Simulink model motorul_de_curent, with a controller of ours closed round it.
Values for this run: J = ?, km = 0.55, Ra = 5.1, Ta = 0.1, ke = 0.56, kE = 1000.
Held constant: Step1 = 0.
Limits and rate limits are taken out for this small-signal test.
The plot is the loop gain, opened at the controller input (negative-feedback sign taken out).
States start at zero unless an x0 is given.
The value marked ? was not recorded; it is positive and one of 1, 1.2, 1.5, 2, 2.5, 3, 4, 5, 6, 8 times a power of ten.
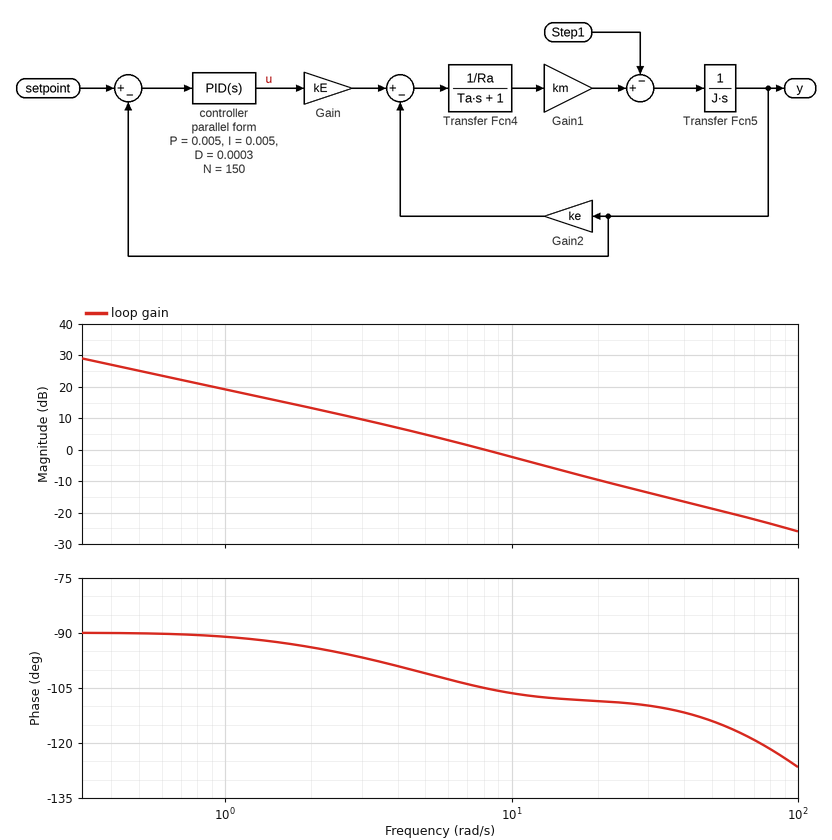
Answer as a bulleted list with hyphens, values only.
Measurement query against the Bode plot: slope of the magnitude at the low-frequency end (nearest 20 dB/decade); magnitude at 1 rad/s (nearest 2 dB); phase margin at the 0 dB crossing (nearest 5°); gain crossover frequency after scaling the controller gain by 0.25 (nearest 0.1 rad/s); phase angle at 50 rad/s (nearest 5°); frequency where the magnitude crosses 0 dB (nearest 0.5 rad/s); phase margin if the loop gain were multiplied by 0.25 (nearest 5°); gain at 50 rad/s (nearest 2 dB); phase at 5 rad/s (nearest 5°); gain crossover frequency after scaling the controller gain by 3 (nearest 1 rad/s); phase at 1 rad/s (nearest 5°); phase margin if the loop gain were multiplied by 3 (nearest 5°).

- -20 dB/decade
- 20 dB
- 75°
- 2.3 rad/s
- -115°
- 8.0 rad/s
- 85°
- -18 dB
- -100°
- 20 rad/s
- -90°
- 70°
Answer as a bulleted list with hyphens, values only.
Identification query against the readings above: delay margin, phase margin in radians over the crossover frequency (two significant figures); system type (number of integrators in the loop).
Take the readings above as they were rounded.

- 0.16 s
- 1
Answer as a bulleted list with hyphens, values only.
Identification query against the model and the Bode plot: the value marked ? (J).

- 0.06
